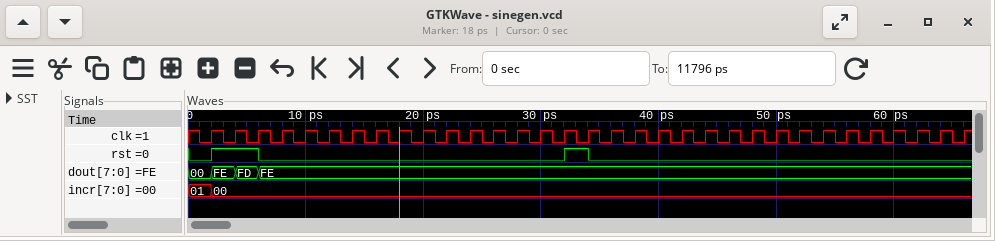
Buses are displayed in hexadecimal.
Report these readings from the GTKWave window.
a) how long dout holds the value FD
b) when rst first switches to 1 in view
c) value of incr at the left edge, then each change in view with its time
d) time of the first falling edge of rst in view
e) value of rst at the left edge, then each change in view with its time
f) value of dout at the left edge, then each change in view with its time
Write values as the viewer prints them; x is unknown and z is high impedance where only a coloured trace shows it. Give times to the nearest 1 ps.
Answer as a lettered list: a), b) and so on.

a) 2 ps
b) 2 ps
c) 01, 00 at 2 ps
d) 6 ps
e) 0, 1 at 2 ps, 0 at 6 ps, 1 at 32 ps, 0 at 34 ps
f) 00, FE at 2 ps, FD at 4 ps, FE at 6 ps
